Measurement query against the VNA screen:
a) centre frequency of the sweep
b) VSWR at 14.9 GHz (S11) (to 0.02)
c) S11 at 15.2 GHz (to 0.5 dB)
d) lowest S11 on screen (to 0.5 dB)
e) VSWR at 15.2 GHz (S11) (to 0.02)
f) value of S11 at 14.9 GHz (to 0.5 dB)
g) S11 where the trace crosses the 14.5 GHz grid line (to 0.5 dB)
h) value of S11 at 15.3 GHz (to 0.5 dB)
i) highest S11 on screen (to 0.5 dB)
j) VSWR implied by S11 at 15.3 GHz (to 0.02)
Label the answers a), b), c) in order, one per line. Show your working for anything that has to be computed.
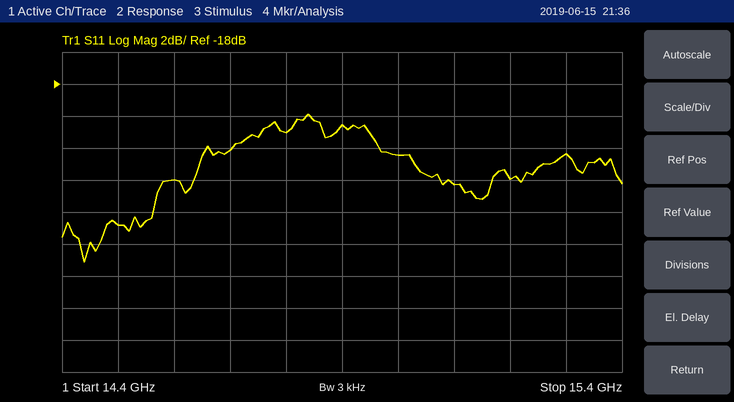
a) 14.9 GHz
b) |Γ| = 10^(-20.5/20) = 0.0944; VSWR = (1 + 0.0944)/(1 − 0.0944) ≈ 1.21, so 1.20 to the nearest 0.02
c) -24.0 dB
d) -29.0 dB
e) |Γ| = 10^(-24/20) = 0.0631; VSWR = (1 + 0.0631)/(1 − 0.0631) ≈ 1.13, so 1.14 to the nearest 0.02
f) -20.5 dB
g) -27.0 dB
h) -22.5 dB
i) -20.0 dB
j) |Γ| = 10^(-22.5/20) = 0.0750; VSWR = (1 + 0.0750)/(1 − 0.0750) ≈ 1.16
